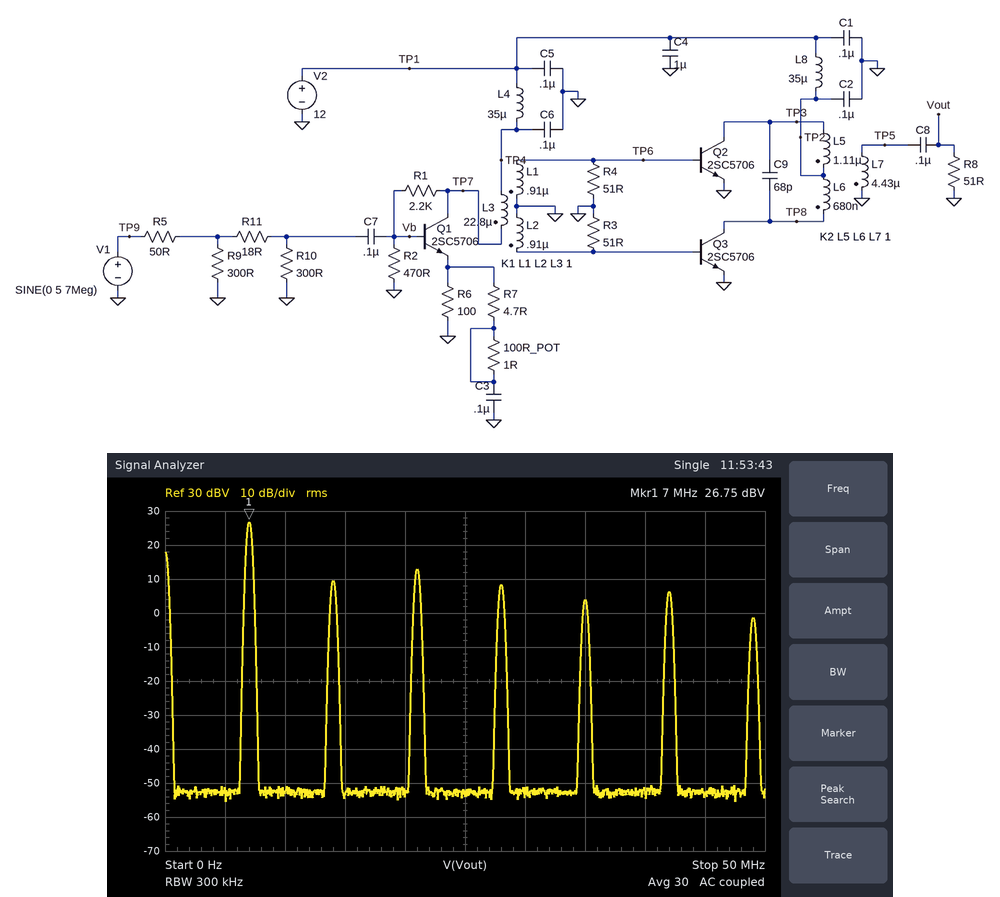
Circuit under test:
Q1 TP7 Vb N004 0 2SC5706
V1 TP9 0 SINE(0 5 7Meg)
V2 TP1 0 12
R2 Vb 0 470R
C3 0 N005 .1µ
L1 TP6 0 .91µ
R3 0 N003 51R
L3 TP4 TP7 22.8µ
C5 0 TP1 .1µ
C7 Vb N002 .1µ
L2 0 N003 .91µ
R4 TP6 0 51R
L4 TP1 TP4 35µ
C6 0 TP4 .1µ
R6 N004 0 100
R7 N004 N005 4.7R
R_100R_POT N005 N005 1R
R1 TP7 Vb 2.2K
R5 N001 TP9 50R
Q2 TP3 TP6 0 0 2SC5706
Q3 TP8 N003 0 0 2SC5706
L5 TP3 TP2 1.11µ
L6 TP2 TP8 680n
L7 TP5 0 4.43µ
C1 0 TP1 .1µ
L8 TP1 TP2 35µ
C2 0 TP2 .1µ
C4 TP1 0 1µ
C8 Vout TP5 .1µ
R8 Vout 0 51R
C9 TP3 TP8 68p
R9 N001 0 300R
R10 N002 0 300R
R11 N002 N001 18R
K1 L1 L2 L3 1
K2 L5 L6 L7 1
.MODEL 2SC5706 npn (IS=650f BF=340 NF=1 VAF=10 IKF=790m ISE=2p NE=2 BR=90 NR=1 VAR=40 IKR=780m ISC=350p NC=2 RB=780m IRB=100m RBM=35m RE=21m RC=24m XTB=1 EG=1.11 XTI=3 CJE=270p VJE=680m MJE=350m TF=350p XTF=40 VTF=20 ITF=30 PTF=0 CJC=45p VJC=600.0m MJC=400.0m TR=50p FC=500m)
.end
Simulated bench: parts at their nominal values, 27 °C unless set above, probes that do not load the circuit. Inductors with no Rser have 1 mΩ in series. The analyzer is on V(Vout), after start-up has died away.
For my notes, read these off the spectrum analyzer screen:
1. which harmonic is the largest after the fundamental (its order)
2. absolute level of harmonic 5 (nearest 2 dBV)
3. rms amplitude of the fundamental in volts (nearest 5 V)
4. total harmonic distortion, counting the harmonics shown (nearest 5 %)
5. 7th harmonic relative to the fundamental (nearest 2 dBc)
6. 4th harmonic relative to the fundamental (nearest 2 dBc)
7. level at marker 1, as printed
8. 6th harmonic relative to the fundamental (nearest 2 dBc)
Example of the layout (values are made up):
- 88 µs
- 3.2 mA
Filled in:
- 3
- 4 dBV
- 20 V
- 30 %
- -28 dBc
- -18 dBc
- 26.75 dBV
- -20 dBc
